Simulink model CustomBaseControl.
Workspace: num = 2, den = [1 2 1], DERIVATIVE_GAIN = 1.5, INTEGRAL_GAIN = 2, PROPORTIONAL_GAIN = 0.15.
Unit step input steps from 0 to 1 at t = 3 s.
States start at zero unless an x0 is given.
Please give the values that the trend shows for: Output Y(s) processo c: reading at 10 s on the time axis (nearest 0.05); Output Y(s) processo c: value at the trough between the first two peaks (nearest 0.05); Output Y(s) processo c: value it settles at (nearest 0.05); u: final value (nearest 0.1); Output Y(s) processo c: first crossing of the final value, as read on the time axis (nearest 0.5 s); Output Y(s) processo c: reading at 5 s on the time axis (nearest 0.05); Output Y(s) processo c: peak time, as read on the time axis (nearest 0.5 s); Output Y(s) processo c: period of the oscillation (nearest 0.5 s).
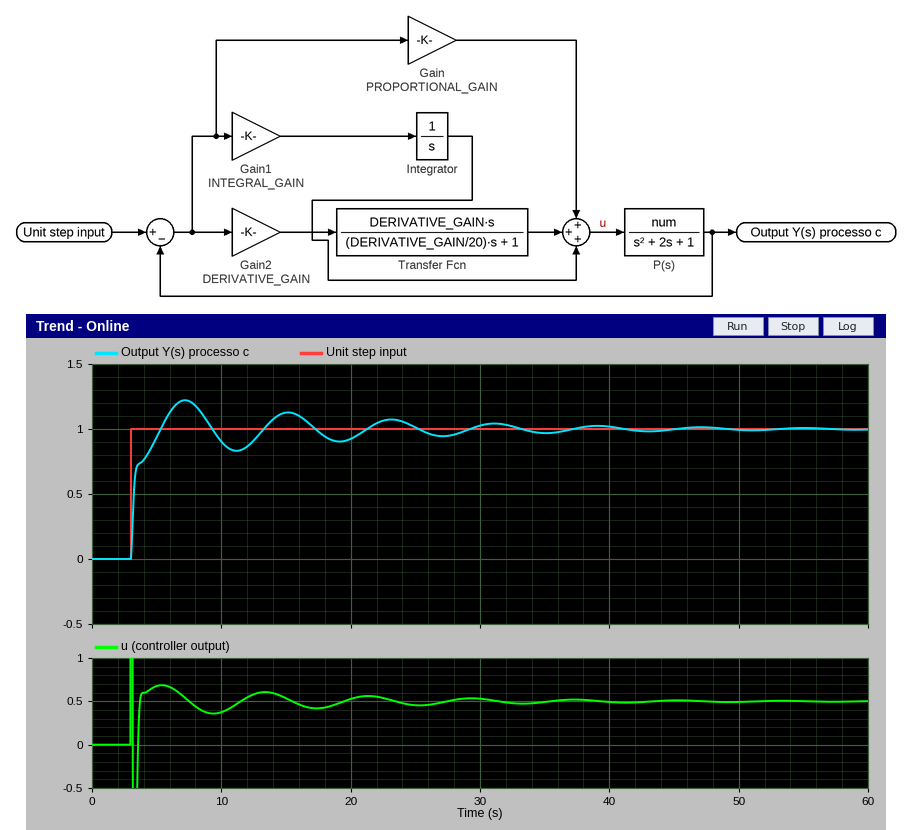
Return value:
0.90
0.85
1.00
0.5
5.5 s
0.95
7.0 s
8.0 s
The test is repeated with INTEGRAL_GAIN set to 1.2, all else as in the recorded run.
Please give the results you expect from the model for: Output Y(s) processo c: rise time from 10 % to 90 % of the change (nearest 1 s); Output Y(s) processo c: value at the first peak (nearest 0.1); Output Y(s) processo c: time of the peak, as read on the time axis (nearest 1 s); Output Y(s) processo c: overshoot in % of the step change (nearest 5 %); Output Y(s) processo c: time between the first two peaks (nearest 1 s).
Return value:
3 s
1.2
9 s
20 %
10 s
